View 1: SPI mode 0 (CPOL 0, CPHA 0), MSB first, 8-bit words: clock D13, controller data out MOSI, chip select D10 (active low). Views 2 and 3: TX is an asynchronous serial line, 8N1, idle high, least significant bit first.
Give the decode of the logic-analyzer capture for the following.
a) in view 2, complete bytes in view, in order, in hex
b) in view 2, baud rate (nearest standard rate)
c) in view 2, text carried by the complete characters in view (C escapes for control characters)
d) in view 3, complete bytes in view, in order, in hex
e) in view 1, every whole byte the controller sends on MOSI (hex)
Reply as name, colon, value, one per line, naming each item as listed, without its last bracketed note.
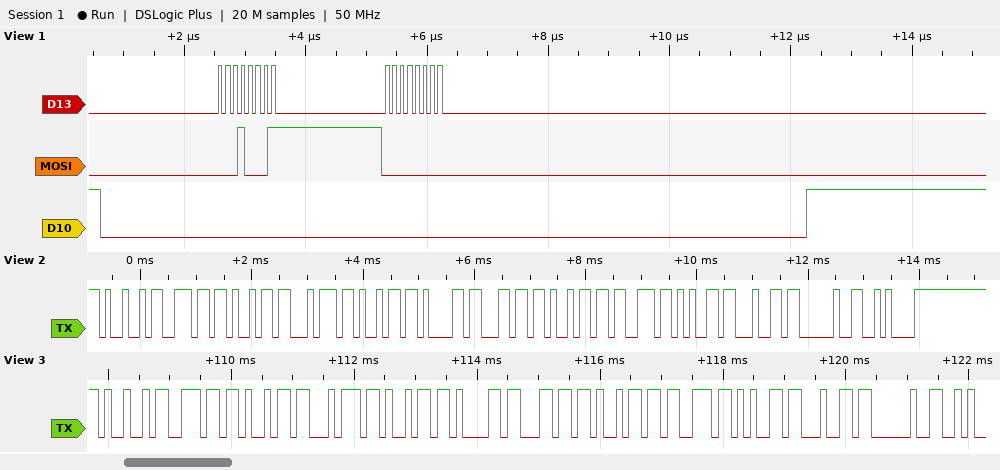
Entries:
in view 2, complete bytes in view, in order, in hex: 49 6E 69 74 69 61 6C 69 73 65 64 20 0A
in view 2, baud rate: 9600 baud
in view 2, text carried by the complete characters in view: "Initialised \n"
in view 3, complete bytes in view, in order, in hex: 49 6E 69 74 69 61 6C 69 73 65 64 20
in view 1, every whole byte the controller sends on MOSI: 11 00
